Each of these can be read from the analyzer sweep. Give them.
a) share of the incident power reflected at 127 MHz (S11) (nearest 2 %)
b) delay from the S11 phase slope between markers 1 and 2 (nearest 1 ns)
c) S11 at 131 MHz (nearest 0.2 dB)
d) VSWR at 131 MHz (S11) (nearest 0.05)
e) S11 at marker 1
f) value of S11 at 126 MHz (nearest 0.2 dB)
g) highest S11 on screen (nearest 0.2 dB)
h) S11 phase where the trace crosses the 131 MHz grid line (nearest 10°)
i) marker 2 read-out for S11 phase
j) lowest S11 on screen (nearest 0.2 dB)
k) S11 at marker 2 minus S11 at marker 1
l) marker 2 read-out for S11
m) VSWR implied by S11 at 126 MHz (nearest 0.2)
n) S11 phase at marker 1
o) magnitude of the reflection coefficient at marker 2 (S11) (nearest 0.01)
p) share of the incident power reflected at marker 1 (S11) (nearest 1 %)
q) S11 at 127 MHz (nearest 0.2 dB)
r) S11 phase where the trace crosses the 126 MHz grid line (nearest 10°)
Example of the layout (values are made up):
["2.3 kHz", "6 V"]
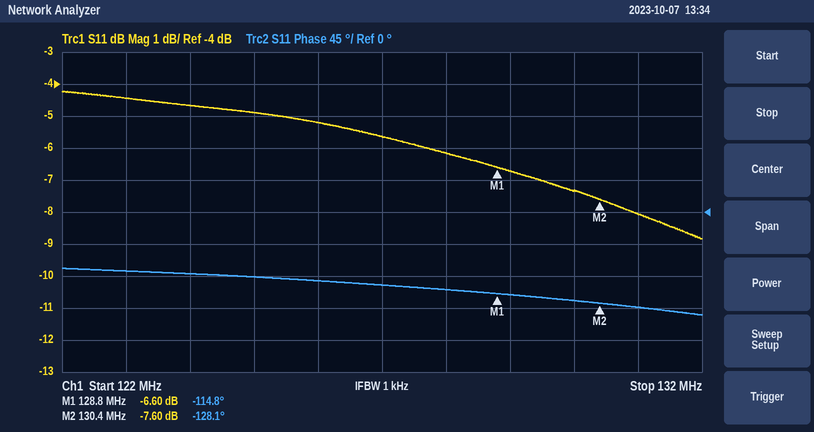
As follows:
["28 %", "23 ns", "-8.0 dB", "2.30", "-6.60 dB", "-5.2 dB", "-4.2 dB", "-130°", "-128.1°", "-8.8 dB", "-1.00 dB", "-7.60 dB", "3.4", "-114.8°", "0.42", "22 %", "-5.6 dB", "-100°"]
